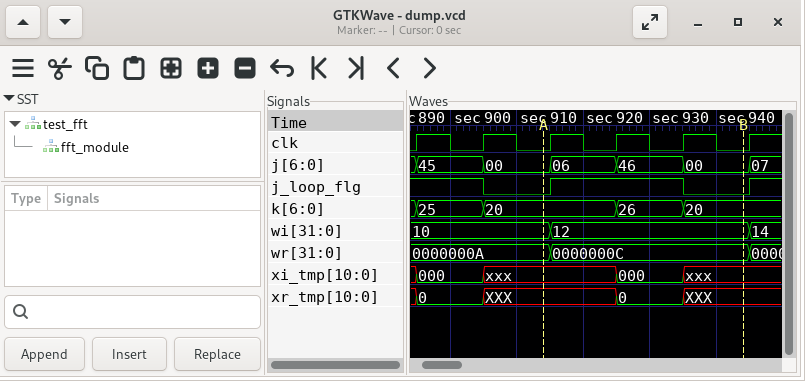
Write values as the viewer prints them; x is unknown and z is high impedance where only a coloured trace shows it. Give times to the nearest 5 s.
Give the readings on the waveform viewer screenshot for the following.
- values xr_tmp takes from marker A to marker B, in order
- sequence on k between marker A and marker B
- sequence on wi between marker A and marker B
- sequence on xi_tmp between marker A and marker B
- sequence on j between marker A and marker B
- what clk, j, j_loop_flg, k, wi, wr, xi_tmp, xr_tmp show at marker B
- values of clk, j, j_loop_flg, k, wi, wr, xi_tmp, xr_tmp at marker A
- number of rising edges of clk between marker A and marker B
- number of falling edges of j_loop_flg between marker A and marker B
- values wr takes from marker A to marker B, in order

XXX, 0, XXX
20, 26, 20
10, 12
xxx, 000, xxx
00, 06, 46, 00
clk=0, j=00, j_loop_flg=0, k=20, wi=12, wr=0000000C, xi_tmp=xxx, xr_tmp=XXX
clk=0, j=00, j_loop_flg=0, k=20, wi=10, wr=0000000A, xi_tmp=xxx, xr_tmp=XXX
3
1
0000000A, 0000000C
